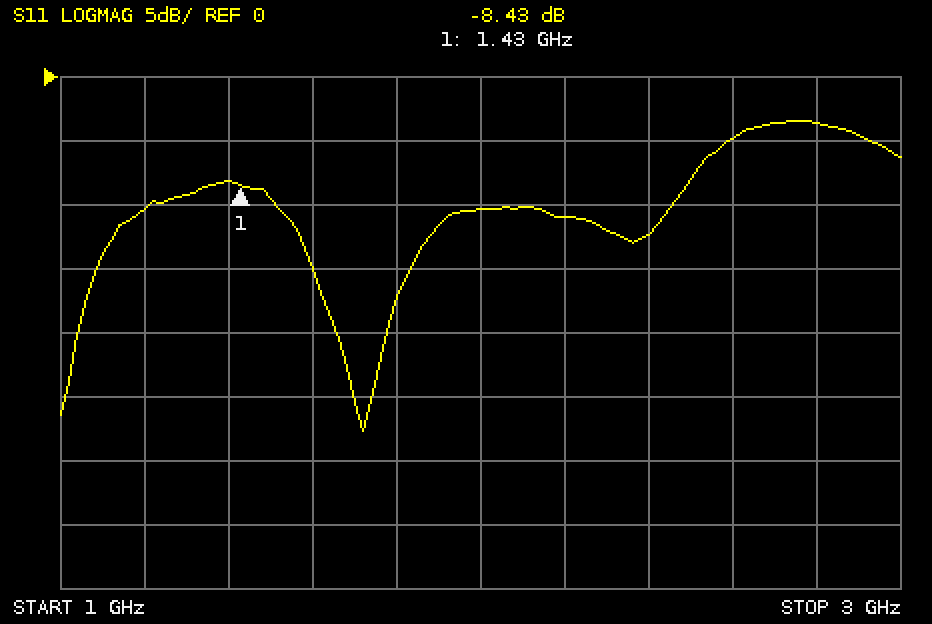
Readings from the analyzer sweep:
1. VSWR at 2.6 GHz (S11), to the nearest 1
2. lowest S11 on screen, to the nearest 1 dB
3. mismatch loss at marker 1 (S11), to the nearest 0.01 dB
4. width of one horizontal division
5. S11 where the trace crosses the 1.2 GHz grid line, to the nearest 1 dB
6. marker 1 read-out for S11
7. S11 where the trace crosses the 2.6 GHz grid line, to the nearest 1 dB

4
-28 dB
0.67 dB
200 MHz
-10 dB
-8.43 dB
-5 dB
